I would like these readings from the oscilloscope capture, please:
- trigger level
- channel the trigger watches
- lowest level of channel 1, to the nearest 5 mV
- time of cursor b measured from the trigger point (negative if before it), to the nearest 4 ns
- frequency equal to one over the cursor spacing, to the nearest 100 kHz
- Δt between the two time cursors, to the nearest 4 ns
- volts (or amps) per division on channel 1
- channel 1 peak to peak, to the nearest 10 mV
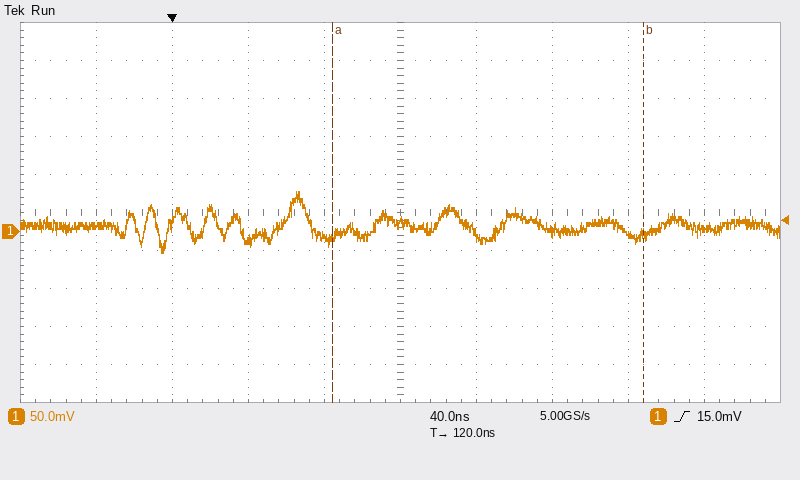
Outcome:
15.0 mV
channel 1
-30 mV
+248 ns
6.1 MHz
164 ns
50 mV
80 mV
